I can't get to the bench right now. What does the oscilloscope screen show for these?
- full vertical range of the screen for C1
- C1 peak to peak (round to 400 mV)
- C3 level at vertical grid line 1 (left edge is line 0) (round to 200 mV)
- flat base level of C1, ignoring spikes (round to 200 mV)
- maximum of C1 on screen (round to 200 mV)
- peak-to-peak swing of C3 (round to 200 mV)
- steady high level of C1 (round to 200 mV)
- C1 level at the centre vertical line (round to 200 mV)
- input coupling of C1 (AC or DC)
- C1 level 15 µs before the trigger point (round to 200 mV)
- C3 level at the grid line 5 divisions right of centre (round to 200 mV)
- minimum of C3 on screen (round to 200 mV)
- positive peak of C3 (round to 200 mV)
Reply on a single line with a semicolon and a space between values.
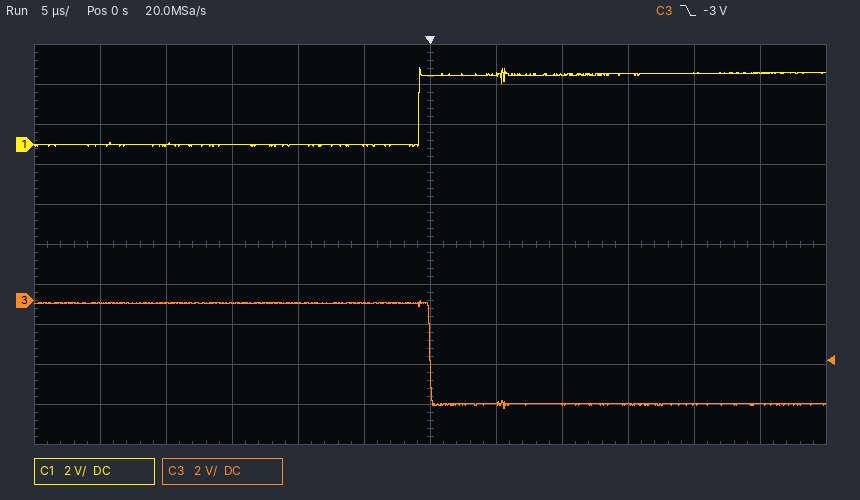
20 V; 4.0 V; -200 mV; 0.0 V; 3.8 V; 5.4 V; 3.6 V; 3.4 V; DC; 0.0 V; -5.2 V; -5.4 V; 0.0 V
